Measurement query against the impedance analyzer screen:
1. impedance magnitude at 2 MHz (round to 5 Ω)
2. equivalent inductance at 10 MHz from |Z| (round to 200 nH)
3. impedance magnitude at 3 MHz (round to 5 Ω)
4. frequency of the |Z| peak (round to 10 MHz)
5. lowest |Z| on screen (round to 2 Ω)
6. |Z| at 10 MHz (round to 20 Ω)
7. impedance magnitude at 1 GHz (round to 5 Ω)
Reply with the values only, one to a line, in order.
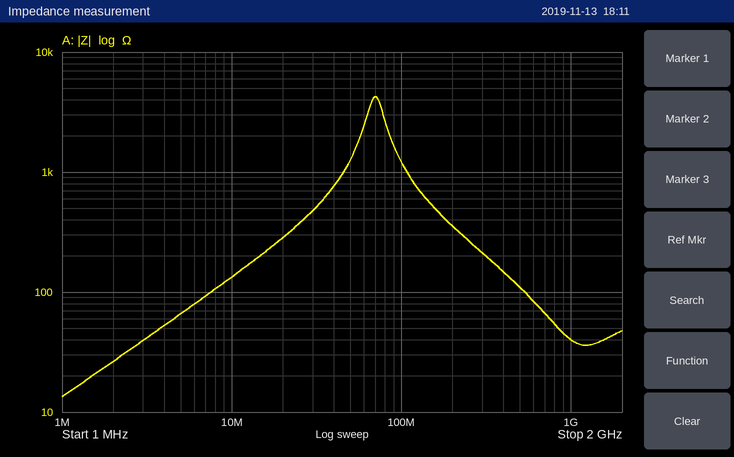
25 Ω
2.2 µH
40 Ω
70 MHz
14 Ω
140 Ω
40 Ω
